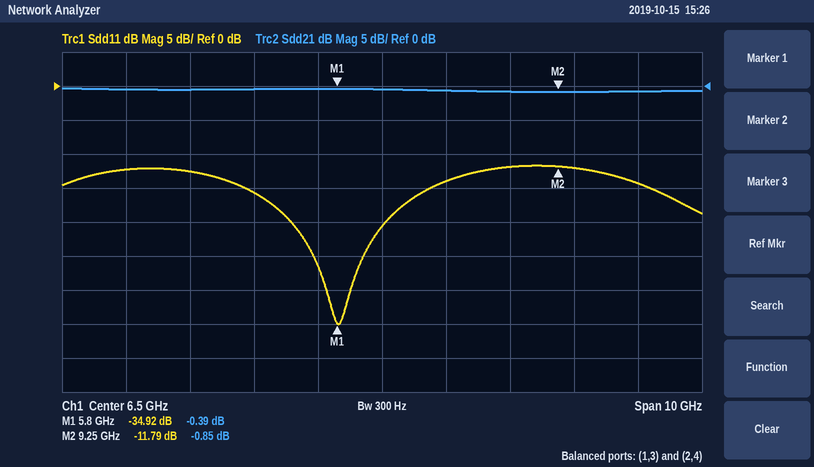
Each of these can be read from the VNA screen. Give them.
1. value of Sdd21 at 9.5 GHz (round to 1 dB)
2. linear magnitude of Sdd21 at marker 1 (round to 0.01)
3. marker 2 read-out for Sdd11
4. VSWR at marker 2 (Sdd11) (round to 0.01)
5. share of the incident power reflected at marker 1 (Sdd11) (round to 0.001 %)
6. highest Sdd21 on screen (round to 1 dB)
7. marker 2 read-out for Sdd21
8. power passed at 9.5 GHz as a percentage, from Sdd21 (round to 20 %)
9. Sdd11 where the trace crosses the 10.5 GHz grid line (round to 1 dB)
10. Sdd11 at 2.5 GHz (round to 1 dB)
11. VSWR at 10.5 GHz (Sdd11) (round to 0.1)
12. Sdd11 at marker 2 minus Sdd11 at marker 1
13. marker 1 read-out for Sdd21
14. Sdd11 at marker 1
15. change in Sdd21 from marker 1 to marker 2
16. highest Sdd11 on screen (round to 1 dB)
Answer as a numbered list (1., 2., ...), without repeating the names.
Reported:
1. -1 dB
2. 0.96
3. -11.79 dB
4. 1.69
5. 0.032 %
6. 0 dB
7. -0.85 dB
8. 80 %
9. -14 dB
10. -12 dB
11. 1.5
12. 23.13 dB
13. -0.39 dB
14. -34.92 dB
15. -0.46 dB
16. -12 dB
